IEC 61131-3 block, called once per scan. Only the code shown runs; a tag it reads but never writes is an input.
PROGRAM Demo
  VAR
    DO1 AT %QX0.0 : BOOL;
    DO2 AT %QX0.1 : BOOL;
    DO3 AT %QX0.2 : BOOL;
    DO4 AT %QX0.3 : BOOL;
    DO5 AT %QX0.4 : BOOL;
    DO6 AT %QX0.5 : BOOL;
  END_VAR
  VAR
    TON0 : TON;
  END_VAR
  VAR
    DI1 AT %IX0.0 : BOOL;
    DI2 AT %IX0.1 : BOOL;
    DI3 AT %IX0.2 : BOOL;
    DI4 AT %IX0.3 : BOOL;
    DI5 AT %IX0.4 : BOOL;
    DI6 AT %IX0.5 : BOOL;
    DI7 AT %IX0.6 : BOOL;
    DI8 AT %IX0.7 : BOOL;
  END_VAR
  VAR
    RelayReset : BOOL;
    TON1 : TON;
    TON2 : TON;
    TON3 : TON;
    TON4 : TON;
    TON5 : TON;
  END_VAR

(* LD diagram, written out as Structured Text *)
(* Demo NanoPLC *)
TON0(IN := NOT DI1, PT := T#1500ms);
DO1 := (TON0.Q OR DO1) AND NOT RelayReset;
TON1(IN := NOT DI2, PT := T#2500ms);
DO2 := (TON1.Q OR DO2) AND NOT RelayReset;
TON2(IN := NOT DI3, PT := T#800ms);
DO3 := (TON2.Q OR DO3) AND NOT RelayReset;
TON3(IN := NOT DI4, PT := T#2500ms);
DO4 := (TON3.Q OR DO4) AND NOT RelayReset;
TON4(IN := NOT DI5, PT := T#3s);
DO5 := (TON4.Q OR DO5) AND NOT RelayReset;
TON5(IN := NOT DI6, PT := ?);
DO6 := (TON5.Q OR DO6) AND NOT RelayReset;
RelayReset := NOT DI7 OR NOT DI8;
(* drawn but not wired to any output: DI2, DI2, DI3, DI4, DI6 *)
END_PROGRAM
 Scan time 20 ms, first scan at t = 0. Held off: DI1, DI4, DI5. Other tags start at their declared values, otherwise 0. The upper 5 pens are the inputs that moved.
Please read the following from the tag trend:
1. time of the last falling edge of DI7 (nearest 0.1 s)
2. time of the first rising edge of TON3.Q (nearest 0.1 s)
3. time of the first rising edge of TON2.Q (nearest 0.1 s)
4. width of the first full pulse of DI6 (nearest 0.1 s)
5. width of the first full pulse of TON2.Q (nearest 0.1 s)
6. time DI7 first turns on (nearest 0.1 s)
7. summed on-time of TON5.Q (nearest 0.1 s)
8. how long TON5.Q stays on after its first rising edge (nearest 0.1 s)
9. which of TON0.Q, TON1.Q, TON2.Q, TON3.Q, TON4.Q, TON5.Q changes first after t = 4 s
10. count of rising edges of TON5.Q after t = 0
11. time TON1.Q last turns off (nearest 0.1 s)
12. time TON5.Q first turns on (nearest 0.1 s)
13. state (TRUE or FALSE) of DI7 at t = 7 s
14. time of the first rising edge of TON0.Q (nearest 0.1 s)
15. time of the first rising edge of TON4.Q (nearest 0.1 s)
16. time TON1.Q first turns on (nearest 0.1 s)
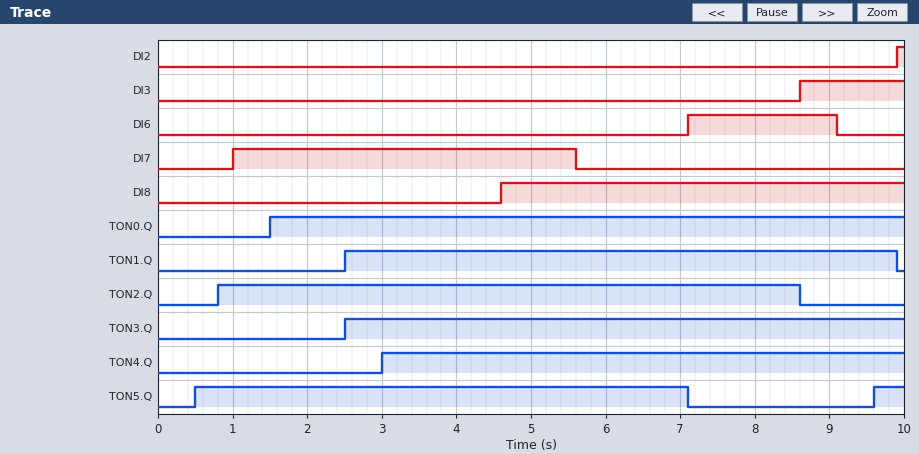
5.6 s
2.5 s
0.8 s
2.0 s
7.8 s
1.0 s
7.0 s
6.6 s
TON5.Q
2
9.9 s
0.5 s
FALSE
1.5 s
3.0 s
2.5 s
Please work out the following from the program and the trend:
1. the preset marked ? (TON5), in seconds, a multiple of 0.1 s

0.5 s
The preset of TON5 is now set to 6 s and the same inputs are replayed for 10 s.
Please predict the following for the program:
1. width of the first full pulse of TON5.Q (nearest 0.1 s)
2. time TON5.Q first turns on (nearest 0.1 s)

1.1 s
6.0 s
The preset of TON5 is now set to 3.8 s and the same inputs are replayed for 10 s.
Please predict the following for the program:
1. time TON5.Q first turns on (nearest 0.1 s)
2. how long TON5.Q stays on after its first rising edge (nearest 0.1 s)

3.8 s
3.3 s
